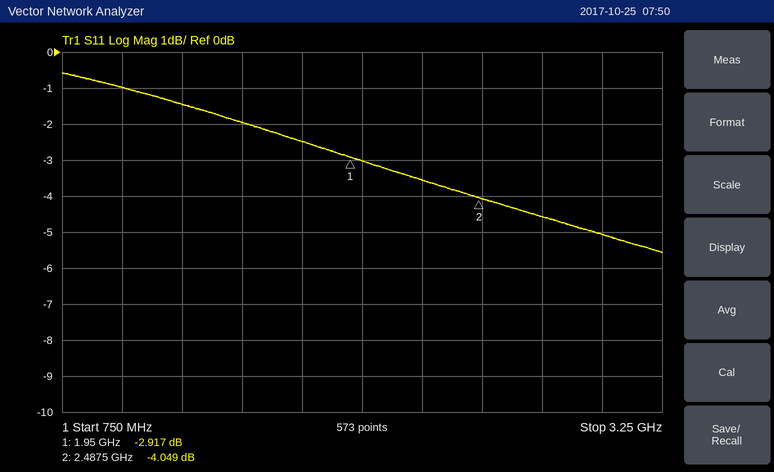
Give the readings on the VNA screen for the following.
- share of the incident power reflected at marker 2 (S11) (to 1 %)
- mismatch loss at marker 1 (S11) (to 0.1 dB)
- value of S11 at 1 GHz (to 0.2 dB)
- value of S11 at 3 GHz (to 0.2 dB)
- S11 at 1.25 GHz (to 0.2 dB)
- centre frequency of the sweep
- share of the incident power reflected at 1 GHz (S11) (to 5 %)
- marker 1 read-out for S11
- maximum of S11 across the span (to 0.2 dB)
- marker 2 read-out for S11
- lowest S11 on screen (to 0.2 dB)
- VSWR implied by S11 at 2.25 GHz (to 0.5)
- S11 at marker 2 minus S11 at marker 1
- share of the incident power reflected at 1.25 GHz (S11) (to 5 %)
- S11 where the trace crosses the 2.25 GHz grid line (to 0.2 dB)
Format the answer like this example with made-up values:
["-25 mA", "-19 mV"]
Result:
["39 %", "3.1 dB", "-1.0 dB", "-5.0 dB", "-1.4 dB", "2 GHz", "80 %", "-2.917 dB", "-0.6 dB", "-4.049 dB", "-5.6 dB", "5.0", "-1.132 dB", "70 %", "-3.6 dB"]
